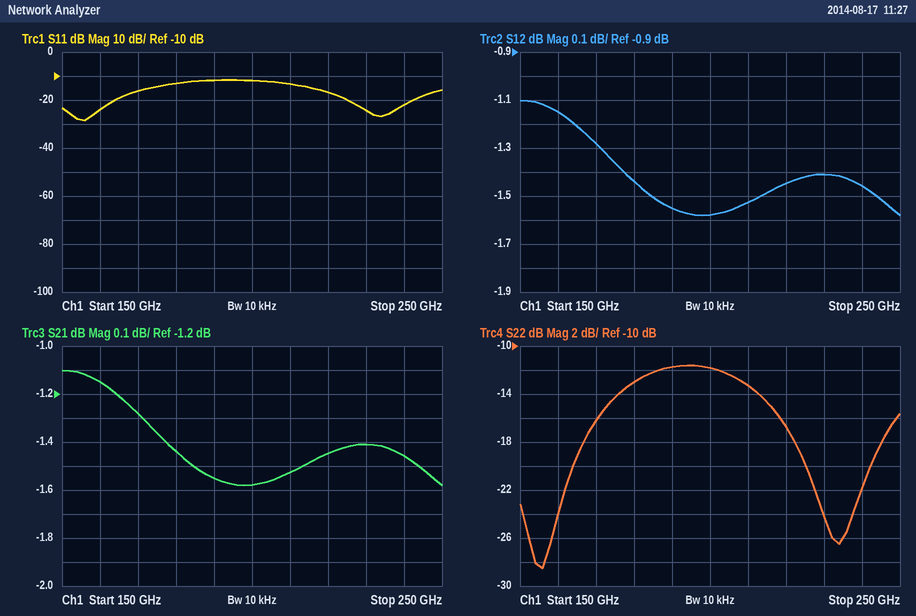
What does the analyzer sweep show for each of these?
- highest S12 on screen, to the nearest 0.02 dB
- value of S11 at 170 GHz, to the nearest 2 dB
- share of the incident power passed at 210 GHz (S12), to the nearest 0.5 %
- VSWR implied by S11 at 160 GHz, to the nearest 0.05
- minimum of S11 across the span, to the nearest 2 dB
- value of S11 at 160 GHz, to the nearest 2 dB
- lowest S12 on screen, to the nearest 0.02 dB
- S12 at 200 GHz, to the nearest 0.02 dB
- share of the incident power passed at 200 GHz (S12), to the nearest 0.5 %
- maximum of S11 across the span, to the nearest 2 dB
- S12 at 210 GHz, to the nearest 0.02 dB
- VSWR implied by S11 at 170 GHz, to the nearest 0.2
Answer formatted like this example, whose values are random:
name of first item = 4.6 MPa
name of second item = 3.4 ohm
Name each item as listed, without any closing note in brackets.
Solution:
highest S12 on screen, to the nearest 0.02 dB = -1.10 dB
value of S11 at 170 GHz, to the nearest 2 dB = -16 dB
share of the incident power passed at 210 GHz (S12), to the nearest 0.5 % = 70.5 %
VSWR implied by S11 at 160 GHz, to the nearest 0.05 = 1.15
minimum of S11 across the span, to the nearest 2 dB = -28 dB
value of S11 at 160 GHz, to the nearest 2 dB = -24 dB
lowest S12 on screen, to the nearest 0.02 dB = -1.58 dB
S12 at 200 GHz, to the nearest 0.02 dB = -1.58 dB
share of the incident power passed at 200 GHz (S12), to the nearest 0.5 % = 69.5 %
maximum of S11 across the span, to the nearest 2 dB = -12 dB
S12 at 210 GHz, to the nearest 0.02 dB = -1.52 dB
VSWR implied by S11 at 170 GHz, to the nearest 0.2 = 1.4
